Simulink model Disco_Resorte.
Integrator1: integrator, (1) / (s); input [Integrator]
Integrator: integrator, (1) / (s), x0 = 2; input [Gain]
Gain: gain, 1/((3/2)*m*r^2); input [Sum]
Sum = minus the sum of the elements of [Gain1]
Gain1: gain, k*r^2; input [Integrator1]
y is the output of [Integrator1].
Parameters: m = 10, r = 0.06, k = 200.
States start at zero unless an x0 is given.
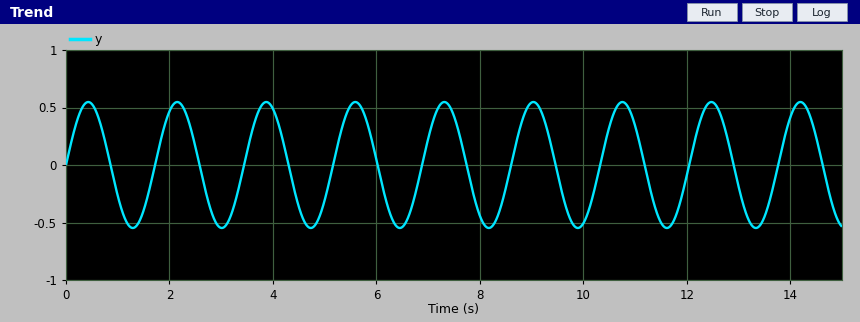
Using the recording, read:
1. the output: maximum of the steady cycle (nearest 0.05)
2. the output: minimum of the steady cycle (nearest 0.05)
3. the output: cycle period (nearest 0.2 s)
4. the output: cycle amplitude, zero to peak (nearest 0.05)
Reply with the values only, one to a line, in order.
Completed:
0.55
-0.55
1.8 s
0.55
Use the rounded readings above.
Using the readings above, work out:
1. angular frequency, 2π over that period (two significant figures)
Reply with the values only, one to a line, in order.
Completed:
3.5 rad/s
